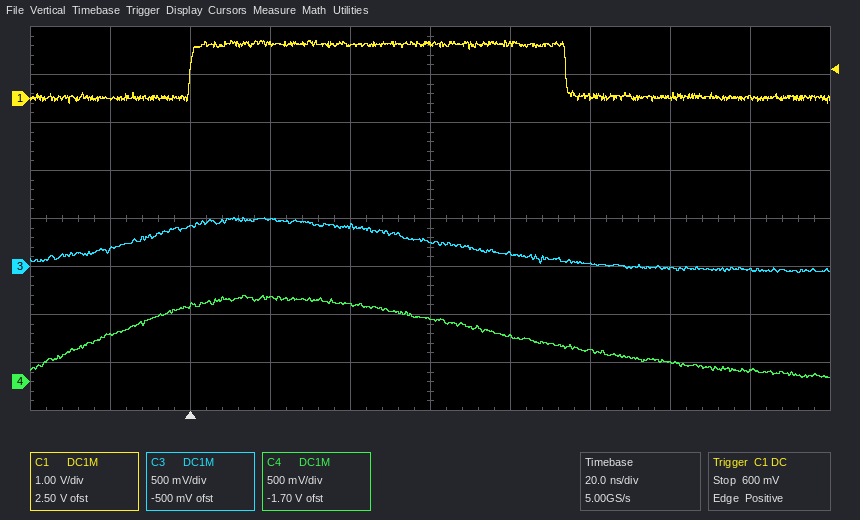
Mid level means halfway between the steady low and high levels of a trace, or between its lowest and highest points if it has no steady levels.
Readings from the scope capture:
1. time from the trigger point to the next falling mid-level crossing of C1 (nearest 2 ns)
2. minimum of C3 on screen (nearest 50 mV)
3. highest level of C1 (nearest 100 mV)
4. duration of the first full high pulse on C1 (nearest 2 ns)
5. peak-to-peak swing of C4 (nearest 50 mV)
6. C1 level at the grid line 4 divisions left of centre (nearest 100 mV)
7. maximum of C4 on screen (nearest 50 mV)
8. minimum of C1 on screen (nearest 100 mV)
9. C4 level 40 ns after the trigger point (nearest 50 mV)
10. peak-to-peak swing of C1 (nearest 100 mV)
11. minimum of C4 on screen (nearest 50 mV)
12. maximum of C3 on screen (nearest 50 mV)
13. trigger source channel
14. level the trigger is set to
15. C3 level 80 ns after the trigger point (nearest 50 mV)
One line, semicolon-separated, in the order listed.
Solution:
94 ns; -50 mV; 1.2 V; 94 ns; 850 mV; 0.0 V; 900 mV; -100 mV; 800 mV; 1.3 V; 50 mV; 500 mV; C1; 600 mV; 150 mV
